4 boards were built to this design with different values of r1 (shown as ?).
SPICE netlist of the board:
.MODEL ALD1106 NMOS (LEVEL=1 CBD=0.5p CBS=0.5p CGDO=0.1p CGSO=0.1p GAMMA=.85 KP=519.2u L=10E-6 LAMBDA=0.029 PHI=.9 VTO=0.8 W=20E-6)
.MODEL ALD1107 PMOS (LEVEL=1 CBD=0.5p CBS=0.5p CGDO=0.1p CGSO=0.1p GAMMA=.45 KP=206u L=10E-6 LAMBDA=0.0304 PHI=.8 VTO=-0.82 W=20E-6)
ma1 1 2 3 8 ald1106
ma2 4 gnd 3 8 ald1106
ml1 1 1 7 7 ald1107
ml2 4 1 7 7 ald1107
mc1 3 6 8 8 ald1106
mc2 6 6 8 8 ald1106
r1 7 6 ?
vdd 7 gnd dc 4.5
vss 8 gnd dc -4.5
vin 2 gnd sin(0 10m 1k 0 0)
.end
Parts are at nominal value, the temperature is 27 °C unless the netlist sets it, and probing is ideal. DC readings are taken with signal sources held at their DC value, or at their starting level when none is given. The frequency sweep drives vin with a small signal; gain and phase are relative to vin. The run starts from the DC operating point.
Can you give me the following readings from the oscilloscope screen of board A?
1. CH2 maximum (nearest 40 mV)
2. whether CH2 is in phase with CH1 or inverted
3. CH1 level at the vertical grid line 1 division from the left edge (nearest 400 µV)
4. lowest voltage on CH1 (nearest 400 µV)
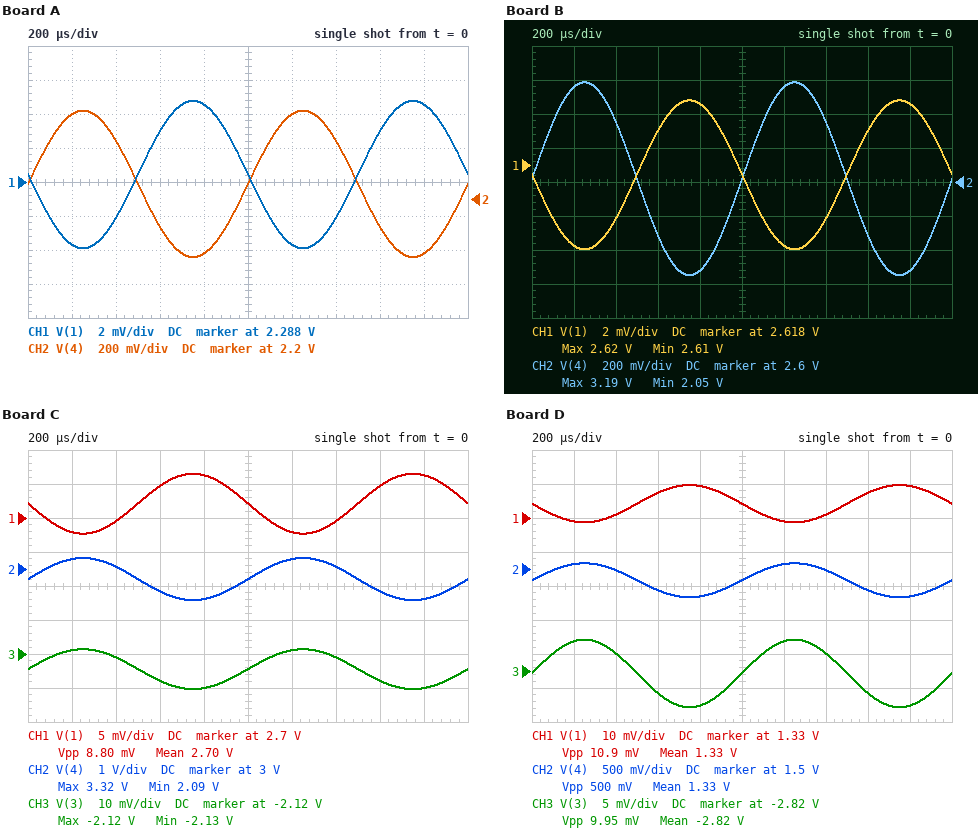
2.72 V
inverted
2.2844 V
2.2840 V
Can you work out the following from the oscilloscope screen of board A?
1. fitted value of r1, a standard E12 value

8.2 kΩ
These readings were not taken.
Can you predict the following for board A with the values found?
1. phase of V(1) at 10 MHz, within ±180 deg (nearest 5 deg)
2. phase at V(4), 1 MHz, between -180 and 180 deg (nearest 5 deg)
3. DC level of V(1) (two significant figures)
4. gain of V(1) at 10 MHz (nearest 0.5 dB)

-165 deg
-5 deg
2.3 V
-3.5 dB
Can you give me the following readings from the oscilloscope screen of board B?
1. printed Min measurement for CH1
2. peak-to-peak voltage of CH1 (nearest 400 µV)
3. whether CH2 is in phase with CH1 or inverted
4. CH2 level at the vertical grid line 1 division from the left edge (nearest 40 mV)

2.61 V
8.8 mV
inverted
3.16 V
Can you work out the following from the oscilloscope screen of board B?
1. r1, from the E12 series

15 kΩ
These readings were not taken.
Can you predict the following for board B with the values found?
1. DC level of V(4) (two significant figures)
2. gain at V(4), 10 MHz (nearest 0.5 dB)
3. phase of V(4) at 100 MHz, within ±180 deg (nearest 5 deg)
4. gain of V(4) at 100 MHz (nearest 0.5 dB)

2.6 V
28.0 dB
-105 deg
8.5 dB
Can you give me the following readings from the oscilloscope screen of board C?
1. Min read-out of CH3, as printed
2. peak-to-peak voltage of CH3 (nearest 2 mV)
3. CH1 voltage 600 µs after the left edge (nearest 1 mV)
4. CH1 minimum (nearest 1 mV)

-2.13 V
12 mV
2.705 V
2.698 V
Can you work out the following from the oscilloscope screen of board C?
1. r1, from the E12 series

18 kΩ
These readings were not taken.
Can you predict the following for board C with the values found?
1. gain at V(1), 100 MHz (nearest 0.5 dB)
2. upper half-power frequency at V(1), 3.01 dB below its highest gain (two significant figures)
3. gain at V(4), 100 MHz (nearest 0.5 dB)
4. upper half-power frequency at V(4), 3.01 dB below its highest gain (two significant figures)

-2.5 dB
280 MHz
7.5 dB
4.1 MHz
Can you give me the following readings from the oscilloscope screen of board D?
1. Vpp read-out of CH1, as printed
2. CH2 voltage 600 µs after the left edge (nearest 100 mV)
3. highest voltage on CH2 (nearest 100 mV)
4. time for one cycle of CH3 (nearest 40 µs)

10.9 mV
1.2 V
1.6 V
1.00 ms
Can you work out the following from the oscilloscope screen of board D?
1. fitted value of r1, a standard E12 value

2.2 kΩ
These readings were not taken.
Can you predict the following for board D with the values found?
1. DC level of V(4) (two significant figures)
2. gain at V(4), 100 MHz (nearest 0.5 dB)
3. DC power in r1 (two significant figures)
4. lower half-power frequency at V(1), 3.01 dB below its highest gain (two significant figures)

1.3 V
16.0 dB
16 mW
11 MHz
